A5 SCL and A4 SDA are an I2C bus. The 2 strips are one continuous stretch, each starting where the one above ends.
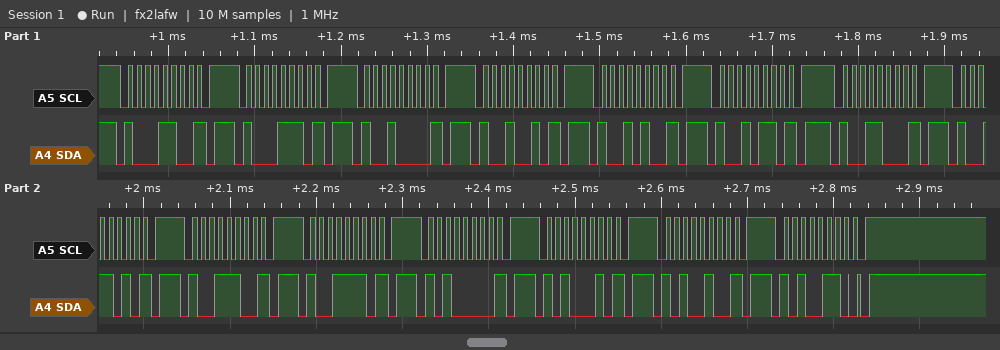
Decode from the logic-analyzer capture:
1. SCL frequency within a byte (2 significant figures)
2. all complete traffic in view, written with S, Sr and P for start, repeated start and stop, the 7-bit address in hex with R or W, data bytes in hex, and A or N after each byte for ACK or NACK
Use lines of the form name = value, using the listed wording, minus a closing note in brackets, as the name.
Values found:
SCL frequency within a byte = 100 kHz
all complete traffic in view, written with S, Sr and P for start, repeated start and stop, the 7-bit address in hex with R or W, data bytes in hex, and A or N after each byte for ACK or NACK = S 46W N P S 47W N P S 48W N P S 49W N P S 4AW N P S 4BW N P S 4CW N P S 4DW N P S 4EW N P S 4FW N P S 50W N P S 51W N P S 52W N P S 53W A P
